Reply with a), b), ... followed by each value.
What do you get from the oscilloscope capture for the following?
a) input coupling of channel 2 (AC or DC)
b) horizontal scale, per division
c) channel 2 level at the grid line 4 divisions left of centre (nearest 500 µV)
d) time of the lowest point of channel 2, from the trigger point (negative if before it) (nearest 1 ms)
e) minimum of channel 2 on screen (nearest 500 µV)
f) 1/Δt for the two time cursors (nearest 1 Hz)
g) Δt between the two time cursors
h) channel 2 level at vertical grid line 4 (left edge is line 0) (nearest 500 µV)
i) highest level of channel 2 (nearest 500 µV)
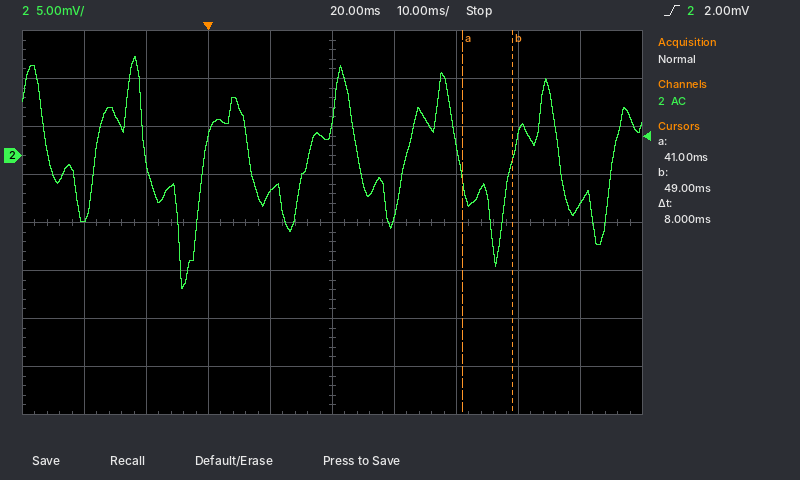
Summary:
a) AC
b) 10 ms
c) -6.5 mV
d) -4 ms
e) -14.0 mV
f) 125 Hz
g) 8 ms
h) -4.0 mV
i) 10.5 mV
